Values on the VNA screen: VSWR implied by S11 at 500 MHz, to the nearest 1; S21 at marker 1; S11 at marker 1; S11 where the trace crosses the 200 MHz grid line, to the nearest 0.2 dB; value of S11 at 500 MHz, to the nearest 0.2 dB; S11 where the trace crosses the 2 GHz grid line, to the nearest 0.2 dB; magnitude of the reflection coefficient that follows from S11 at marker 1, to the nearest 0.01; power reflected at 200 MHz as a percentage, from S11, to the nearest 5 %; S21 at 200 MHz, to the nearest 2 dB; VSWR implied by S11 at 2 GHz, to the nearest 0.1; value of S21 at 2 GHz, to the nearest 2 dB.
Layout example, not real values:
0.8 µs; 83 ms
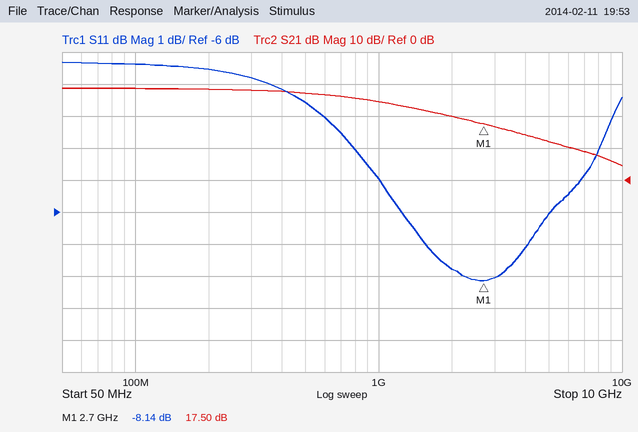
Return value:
7; 17.50 dB; -8.14 dB; -1.6 dB; -2.6 dB; -7.8 dB; 0.39; 70 %; 28 dB; 2.4; 20 dB
